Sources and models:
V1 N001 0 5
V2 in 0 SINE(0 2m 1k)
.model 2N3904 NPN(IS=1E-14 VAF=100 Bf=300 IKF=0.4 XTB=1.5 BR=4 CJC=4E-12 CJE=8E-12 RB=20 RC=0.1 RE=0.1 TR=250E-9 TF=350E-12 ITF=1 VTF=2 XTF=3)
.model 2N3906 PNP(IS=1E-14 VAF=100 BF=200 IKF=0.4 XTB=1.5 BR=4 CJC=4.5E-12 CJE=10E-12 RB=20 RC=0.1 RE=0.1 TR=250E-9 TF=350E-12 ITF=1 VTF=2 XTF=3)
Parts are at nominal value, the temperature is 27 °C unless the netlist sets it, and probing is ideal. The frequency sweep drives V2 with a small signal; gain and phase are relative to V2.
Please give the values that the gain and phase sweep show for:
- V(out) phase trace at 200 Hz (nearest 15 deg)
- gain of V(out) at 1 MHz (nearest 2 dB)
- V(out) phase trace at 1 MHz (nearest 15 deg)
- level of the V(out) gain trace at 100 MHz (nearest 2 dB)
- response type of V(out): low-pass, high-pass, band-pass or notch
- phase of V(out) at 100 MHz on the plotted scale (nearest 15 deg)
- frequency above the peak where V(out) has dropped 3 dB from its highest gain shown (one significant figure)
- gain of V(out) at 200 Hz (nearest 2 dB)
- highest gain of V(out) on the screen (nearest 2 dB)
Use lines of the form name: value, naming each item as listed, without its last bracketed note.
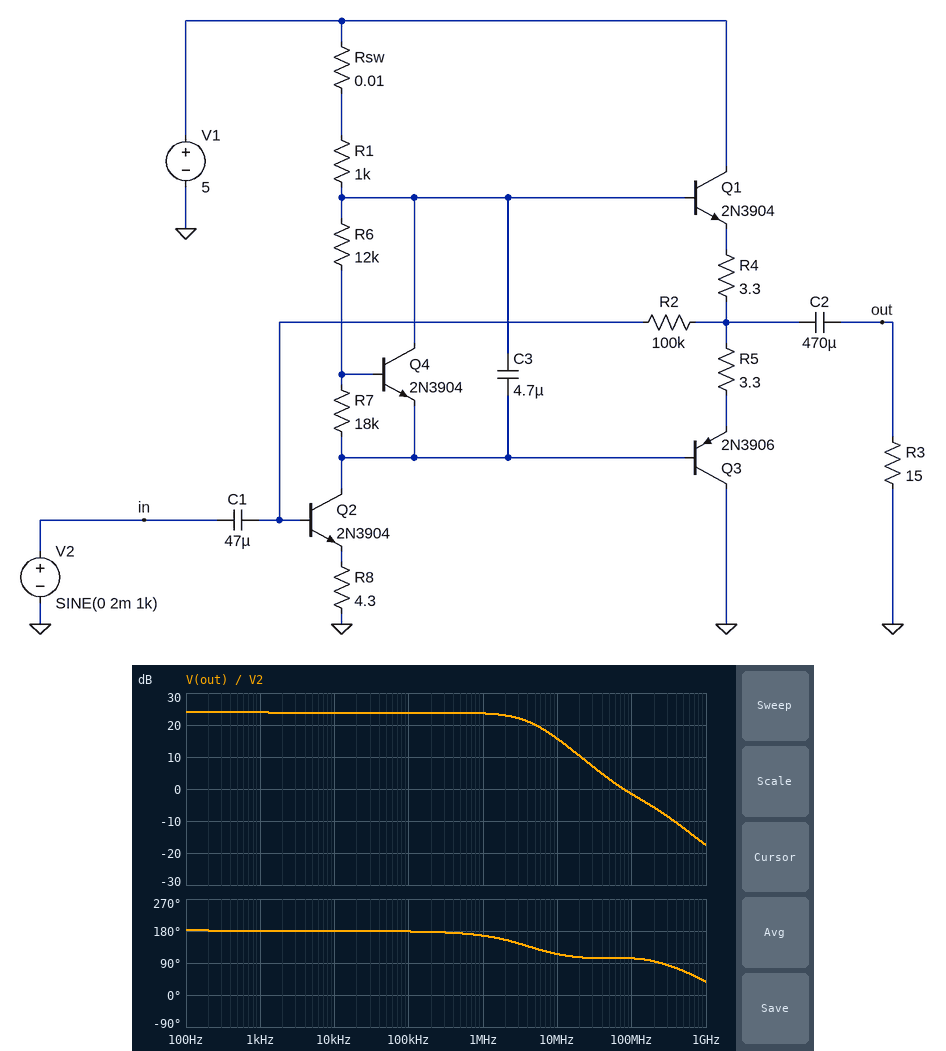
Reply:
V(out) phase trace at 200 Hz: 180 deg
gain of V(out) at 1 MHz: 24 dB
V(out) phase trace at 1 MHz: 165 deg
level of the V(out) gain trace at 100 MHz: -2 dB
response type of V(out): low-pass, high-pass, band-pass or notch: low-pass
phase of V(out) at 100 MHz on the plotted scale: 105 deg
frequency above the peak where V(out) has dropped 3 dB from its highest gain shown: 4 MHz
gain of V(out) at 200 Hz: 24 dB
highest gain of V(out) on the screen: 24 dB
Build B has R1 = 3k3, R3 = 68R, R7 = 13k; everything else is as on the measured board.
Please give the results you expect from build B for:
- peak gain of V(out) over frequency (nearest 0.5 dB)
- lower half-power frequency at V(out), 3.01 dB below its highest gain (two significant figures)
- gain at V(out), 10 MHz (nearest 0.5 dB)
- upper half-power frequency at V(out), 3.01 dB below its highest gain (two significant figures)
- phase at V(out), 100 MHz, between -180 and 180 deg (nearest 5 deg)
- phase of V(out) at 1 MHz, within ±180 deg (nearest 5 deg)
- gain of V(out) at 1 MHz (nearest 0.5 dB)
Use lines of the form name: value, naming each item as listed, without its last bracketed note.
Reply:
peak gain of V(out) over frequency: 37.0 dB
lower half-power frequency at V(out), 3.01 dB below its highest gain: 4.5 Hz
gain at V(out), 10 MHz: 24.5 dB
upper half-power frequency at V(out), 3.01 dB below its highest gain: 2.3 MHz
phase at V(out), 100 MHz, between -180 and 180 deg: 80 deg
phase of V(out) at 1 MHz, within ±180 deg: 155 deg
gain of V(out) at 1 MHz: 36.5 dB
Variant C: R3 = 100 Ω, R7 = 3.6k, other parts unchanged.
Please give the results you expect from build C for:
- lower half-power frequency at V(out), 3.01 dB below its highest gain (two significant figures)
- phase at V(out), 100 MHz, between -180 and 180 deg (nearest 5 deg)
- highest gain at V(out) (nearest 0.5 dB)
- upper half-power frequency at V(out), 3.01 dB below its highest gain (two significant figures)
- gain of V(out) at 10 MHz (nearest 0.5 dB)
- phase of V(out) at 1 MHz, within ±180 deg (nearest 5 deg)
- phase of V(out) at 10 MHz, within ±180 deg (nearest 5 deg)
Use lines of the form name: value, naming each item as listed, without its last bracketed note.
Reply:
lower half-power frequency at V(out), 3.01 dB below its highest gain: 11 Hz
phase at V(out), 100 MHz, between -180 and 180 deg: 45 deg
highest gain at V(out): 33.5 dB
upper half-power frequency at V(out), 3.01 dB below its highest gain: 1.7 MHz
gain of V(out) at 10 MHz: 18.0 dB
phase of V(out) at 1 MHz, within ±180 deg: 150 deg
phase of V(out) at 10 MHz, within ±180 deg: 95 deg
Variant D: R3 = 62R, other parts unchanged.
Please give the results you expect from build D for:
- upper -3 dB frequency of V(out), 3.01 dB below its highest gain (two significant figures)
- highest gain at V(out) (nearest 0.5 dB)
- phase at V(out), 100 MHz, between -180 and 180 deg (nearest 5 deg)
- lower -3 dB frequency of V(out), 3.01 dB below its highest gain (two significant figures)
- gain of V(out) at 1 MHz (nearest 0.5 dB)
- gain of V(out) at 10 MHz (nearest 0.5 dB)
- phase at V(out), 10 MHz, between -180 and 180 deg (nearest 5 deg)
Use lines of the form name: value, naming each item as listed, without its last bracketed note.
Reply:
upper -3 dB frequency of V(out), 3.01 dB below its highest gain: 5.3 MHz
highest gain at V(out): 32.0 dB
phase at V(out), 100 MHz, between -180 and 180 deg: 95 deg
lower -3 dB frequency of V(out), 3.01 dB below its highest gain: 3.7 Hz
gain of V(out) at 1 MHz: 31.5 dB
gain of V(out) at 10 MHz: 25.5 dB
phase at V(out), 10 MHz, between -180 and 180 deg: 120 deg
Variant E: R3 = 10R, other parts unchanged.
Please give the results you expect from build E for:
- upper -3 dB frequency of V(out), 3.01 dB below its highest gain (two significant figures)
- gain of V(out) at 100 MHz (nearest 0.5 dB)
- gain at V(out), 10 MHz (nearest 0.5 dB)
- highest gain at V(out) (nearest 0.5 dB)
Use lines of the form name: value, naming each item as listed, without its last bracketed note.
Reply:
upper -3 dB frequency of V(out), 3.01 dB below its highest gain: 3.8 MHz
gain of V(out) at 100 MHz: -5.0 dB
gain at V(out), 10 MHz: 12.5 dB
highest gain at V(out): 21.0 dB
